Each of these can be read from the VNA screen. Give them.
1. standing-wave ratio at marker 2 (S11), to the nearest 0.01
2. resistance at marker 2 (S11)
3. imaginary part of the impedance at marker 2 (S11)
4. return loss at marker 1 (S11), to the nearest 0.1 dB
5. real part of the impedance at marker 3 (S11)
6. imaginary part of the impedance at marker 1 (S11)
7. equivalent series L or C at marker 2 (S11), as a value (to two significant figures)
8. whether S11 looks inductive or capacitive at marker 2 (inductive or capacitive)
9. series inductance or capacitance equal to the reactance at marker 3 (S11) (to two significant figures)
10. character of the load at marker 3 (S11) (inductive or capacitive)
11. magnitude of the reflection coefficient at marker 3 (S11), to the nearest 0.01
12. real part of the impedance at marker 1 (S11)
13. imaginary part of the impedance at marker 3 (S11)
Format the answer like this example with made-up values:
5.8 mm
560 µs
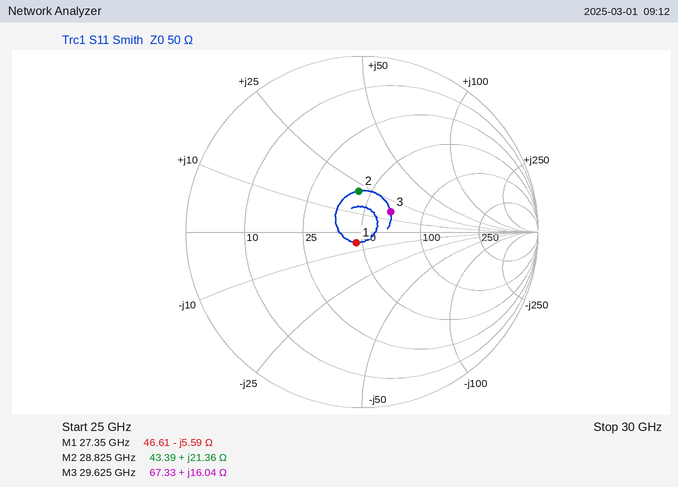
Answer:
1.61
43.39 Ω
+21.36 Ω
23.4 dB
67.33 Ω
-5.59 Ω
120 pH
inductive
86 pH
inductive
0.20
46.61 Ω
+16.04 Ω
